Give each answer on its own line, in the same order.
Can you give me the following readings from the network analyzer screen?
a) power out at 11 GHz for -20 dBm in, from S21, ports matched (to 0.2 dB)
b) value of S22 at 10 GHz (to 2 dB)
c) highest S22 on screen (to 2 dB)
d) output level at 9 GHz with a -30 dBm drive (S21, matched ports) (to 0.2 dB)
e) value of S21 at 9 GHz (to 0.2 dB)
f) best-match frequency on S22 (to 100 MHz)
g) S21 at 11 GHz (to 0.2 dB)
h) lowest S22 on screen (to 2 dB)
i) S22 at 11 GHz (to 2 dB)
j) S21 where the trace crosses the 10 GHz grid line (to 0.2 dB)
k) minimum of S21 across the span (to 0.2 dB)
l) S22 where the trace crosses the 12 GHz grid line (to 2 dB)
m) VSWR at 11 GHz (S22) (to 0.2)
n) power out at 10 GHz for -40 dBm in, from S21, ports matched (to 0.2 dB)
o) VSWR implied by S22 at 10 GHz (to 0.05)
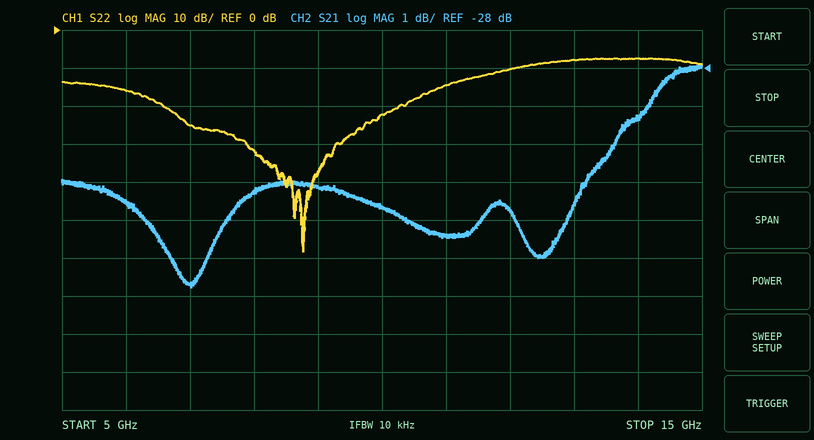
-52.4 dBm
-22 dB
-8 dB
-61.2 dBm
-31.2 dB
8.8 GHz
-32.4 dB
-58 dB
-14 dB
-31.6 dB
-33.8 dB
-10 dB
1.4
-71.6 dBm
1.15
